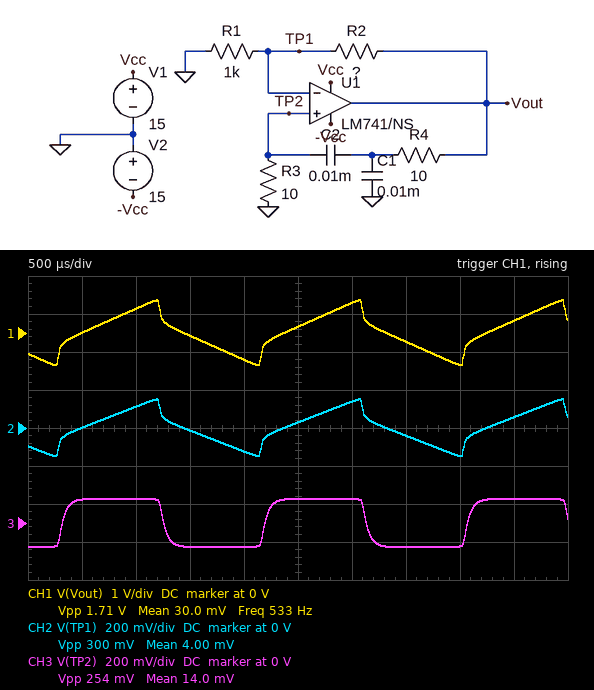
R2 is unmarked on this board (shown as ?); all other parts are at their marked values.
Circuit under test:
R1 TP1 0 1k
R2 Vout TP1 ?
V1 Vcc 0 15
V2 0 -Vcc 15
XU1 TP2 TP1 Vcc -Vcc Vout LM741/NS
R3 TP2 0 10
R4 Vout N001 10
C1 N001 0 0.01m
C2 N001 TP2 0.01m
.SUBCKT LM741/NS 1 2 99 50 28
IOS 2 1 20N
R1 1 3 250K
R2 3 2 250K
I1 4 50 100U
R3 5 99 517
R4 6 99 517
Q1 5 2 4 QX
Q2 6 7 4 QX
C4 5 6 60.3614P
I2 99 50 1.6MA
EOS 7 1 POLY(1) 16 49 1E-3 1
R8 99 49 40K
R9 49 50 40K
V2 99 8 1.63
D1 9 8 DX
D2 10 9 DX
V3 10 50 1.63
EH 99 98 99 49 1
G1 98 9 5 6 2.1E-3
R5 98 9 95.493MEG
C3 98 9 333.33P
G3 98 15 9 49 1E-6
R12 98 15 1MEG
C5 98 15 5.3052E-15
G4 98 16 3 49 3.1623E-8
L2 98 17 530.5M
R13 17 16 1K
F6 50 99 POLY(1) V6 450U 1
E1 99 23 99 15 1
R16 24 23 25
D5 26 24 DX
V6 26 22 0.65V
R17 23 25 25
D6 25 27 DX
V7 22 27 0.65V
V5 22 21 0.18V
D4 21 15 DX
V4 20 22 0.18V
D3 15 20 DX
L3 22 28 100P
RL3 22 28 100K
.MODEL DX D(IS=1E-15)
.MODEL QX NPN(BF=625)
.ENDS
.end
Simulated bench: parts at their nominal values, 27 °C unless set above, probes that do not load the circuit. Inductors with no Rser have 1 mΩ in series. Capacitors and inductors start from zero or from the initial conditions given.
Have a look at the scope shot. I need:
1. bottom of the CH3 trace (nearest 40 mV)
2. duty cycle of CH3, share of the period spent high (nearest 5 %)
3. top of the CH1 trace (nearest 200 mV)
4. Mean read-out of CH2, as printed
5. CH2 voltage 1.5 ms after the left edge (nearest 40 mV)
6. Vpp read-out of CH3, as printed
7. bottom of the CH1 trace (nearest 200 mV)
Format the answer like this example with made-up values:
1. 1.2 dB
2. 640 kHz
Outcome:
1. -120 mV
2. 50 %
3. 800 mV
4. 4.00 mV
5. 0 V
6. 254 mV
7. -800 mV
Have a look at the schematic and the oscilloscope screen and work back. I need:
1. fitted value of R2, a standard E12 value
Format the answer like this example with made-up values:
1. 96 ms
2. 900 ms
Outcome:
1. 4.7 kΩ
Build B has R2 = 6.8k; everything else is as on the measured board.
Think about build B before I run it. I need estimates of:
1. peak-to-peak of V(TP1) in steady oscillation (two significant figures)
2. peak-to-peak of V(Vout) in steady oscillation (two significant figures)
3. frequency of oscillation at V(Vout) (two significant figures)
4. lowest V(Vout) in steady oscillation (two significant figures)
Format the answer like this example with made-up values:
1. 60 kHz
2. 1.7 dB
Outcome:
1. 290 mV
2. 2.3 V
3. 360 Hz
4. -1.1 V
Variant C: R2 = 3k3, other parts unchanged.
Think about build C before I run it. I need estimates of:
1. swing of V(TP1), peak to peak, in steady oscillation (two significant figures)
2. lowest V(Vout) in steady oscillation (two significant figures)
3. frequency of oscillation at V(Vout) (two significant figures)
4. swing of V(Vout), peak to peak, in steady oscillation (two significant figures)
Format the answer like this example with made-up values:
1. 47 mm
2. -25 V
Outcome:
1. 310 mV
2. -660 mV
3. 780 Hz
4. 1.3 V
